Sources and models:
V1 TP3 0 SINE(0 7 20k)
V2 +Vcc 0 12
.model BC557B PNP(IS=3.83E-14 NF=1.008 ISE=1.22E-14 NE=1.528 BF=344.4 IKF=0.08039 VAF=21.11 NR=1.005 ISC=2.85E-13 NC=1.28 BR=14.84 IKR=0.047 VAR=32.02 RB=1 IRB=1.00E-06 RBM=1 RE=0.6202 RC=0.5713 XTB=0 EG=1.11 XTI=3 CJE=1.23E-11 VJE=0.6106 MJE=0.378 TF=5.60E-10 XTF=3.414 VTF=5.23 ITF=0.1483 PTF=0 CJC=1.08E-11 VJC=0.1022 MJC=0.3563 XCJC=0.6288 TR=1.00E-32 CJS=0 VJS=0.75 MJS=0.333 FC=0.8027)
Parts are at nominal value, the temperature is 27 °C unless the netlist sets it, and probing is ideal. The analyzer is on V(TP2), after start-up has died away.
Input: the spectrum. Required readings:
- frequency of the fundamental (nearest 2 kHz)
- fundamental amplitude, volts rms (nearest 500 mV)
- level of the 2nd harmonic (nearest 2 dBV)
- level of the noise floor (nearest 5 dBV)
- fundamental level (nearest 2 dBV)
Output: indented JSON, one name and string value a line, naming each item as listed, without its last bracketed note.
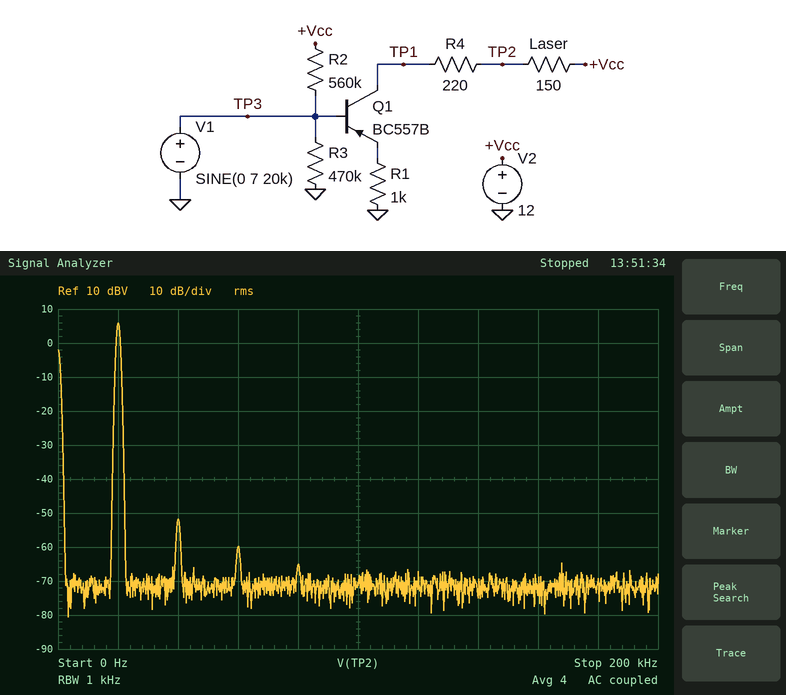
{
  "frequency of the fundamental": "20 kHz",
  "fundamental amplitude, volts rms": "2.0 V",
  "level of the 2nd harmonic": "-52 dBV",
  "level of the noise floor": "-70 dBV",
  "fundamental level": "6 dBV"
}
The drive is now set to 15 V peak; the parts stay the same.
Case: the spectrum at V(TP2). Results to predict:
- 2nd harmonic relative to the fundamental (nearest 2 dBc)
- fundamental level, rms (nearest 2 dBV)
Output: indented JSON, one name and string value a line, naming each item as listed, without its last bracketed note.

{
  "2nd harmonic relative to the fundamental": "-24 dBc",
  "fundamental level, rms": "12 dBV"
}
